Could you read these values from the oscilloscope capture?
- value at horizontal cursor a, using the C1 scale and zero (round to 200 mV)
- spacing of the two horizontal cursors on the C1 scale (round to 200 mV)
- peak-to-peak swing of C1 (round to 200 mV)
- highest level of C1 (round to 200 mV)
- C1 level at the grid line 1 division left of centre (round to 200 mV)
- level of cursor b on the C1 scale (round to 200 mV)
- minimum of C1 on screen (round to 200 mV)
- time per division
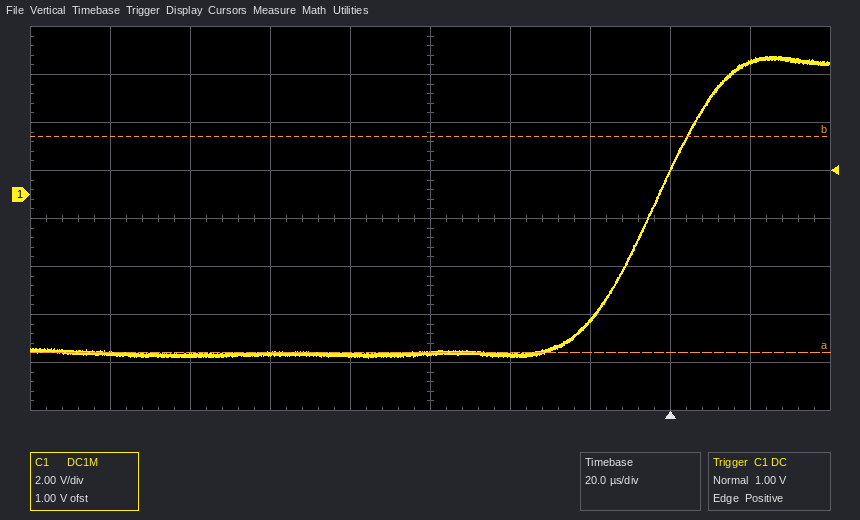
-6.6 V
9.0 V
12.6 V
5.8 V
-6.6 V
2.4 V
-6.8 V
20 µs
